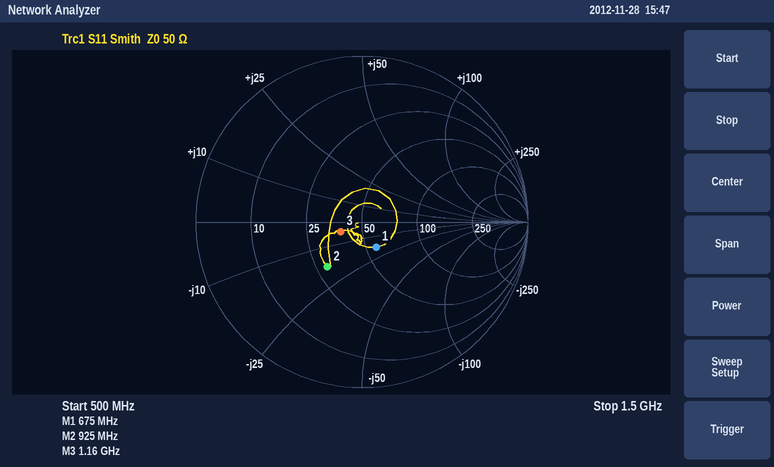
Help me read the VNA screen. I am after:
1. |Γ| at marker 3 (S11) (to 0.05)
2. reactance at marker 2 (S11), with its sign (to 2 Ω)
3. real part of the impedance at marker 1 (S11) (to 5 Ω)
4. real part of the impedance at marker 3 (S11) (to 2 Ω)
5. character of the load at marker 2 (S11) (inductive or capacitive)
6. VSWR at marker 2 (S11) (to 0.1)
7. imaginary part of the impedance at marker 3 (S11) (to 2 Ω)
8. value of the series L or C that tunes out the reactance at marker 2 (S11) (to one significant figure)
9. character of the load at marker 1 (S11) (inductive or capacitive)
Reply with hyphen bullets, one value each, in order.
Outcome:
- 0.15
- -18 Ω
- 55 Ω
- 38 Ω
- capacitive
- 2.0
- -4 Ω
- 3 nH
- capacitive
